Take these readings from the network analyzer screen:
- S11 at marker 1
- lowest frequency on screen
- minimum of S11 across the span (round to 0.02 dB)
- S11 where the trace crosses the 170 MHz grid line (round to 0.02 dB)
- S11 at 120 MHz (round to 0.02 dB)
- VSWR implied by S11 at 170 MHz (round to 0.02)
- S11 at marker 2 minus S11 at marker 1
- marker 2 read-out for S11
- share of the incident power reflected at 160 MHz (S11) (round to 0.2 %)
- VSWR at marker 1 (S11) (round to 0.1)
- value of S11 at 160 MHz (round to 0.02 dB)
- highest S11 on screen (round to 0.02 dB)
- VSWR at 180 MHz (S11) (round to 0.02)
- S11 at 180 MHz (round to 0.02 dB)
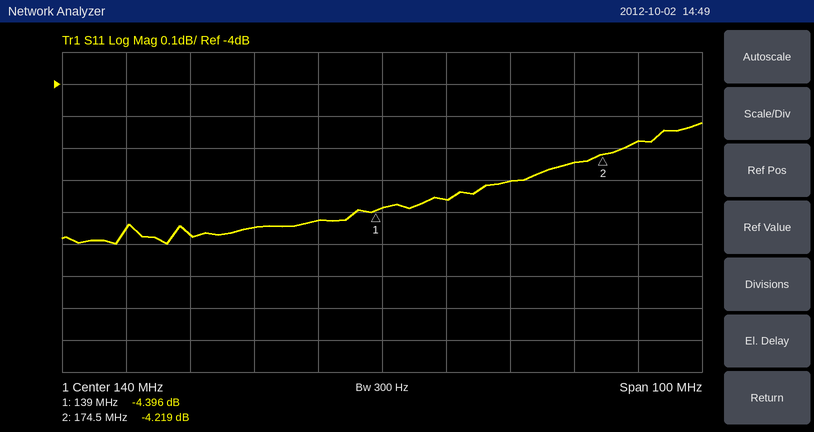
-4.396 dB
90 MHz
-4.50 dB
-4.24 dB
-4.44 dB
4.18
0.177 dB
-4.219 dB
37.2 %
4.0
-4.30 dB
-4.12 dB
4.24
-4.18 dB
